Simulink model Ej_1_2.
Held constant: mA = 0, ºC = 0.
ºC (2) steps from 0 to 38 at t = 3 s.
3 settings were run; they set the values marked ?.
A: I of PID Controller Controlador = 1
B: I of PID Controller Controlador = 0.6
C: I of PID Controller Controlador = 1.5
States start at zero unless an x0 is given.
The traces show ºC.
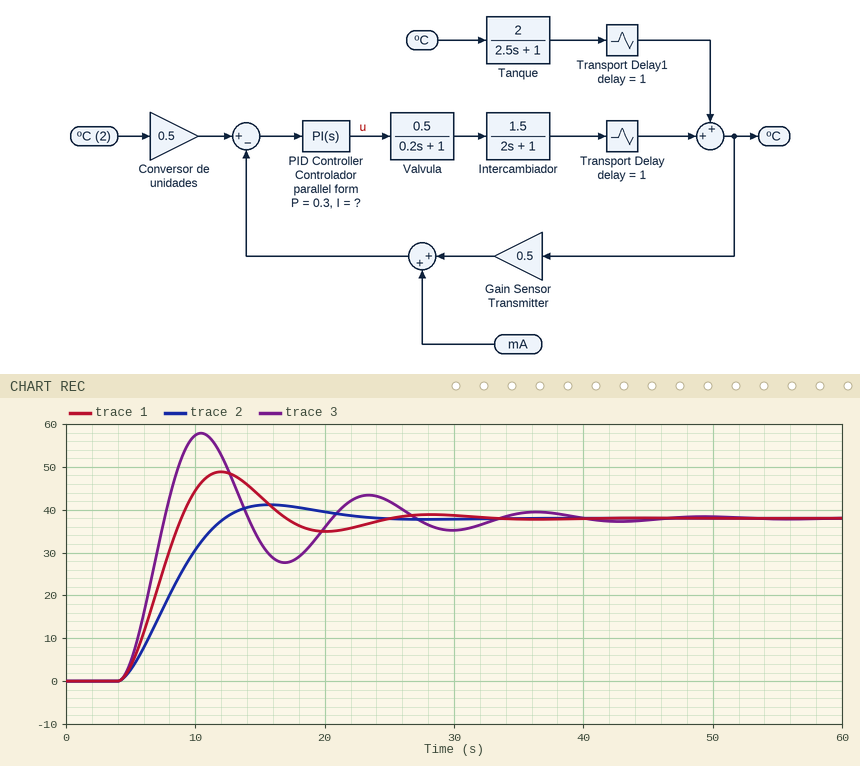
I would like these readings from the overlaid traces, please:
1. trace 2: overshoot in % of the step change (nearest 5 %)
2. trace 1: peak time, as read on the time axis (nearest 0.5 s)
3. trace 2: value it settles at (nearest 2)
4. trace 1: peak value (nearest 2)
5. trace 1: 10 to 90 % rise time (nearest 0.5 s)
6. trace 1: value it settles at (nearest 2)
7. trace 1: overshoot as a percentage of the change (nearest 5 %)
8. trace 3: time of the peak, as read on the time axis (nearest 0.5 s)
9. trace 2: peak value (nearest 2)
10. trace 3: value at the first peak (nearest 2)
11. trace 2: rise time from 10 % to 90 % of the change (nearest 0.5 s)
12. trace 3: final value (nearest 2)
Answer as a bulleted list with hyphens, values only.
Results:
- 10 %
- 12.0 s
- 38
- 48
- 3.5 s
- 38
- 30 %
- 10.5 s
- 42
- 58
- 5.5 s
- 38
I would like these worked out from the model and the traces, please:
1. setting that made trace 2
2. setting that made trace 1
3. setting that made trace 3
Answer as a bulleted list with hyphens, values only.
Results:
- B
- A
- C
